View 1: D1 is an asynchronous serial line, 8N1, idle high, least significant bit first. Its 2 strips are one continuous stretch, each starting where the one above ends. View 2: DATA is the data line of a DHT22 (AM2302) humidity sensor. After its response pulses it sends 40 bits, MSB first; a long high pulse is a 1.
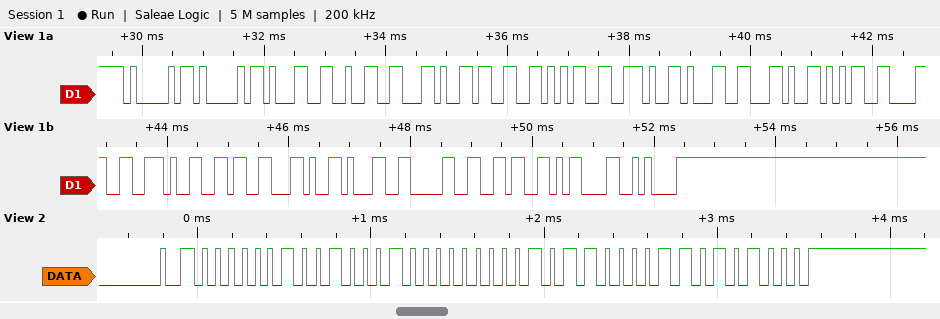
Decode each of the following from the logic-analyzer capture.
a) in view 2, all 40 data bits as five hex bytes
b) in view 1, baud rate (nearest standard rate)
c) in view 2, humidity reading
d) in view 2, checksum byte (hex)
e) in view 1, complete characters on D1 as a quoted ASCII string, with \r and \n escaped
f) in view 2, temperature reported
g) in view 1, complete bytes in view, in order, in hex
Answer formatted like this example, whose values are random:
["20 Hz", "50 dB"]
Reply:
["02 44 01 61 A8", "9600 baud", "58.0 %", "0xA8", "\"AA12,35.1,58.6,106\\r\\n\"", "35.3 °C", "41 41 31 32 2C 33 35 2E 31 2C 35 38 2E 36 2C 31 30 36 0D 0A"]
